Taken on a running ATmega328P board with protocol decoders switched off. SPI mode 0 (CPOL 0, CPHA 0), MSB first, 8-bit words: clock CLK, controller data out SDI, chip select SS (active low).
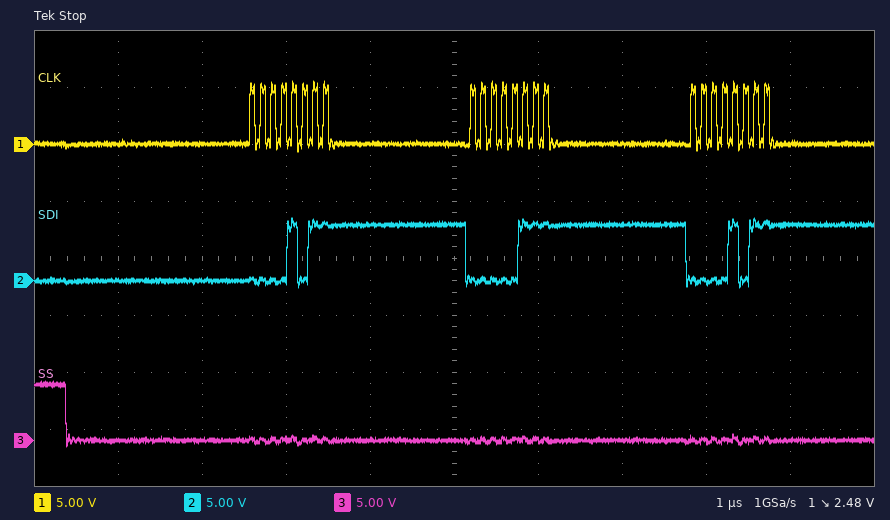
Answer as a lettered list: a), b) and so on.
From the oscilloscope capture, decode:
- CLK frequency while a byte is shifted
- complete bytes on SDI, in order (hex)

a) 8 MHz
b) 0B 07 0B
